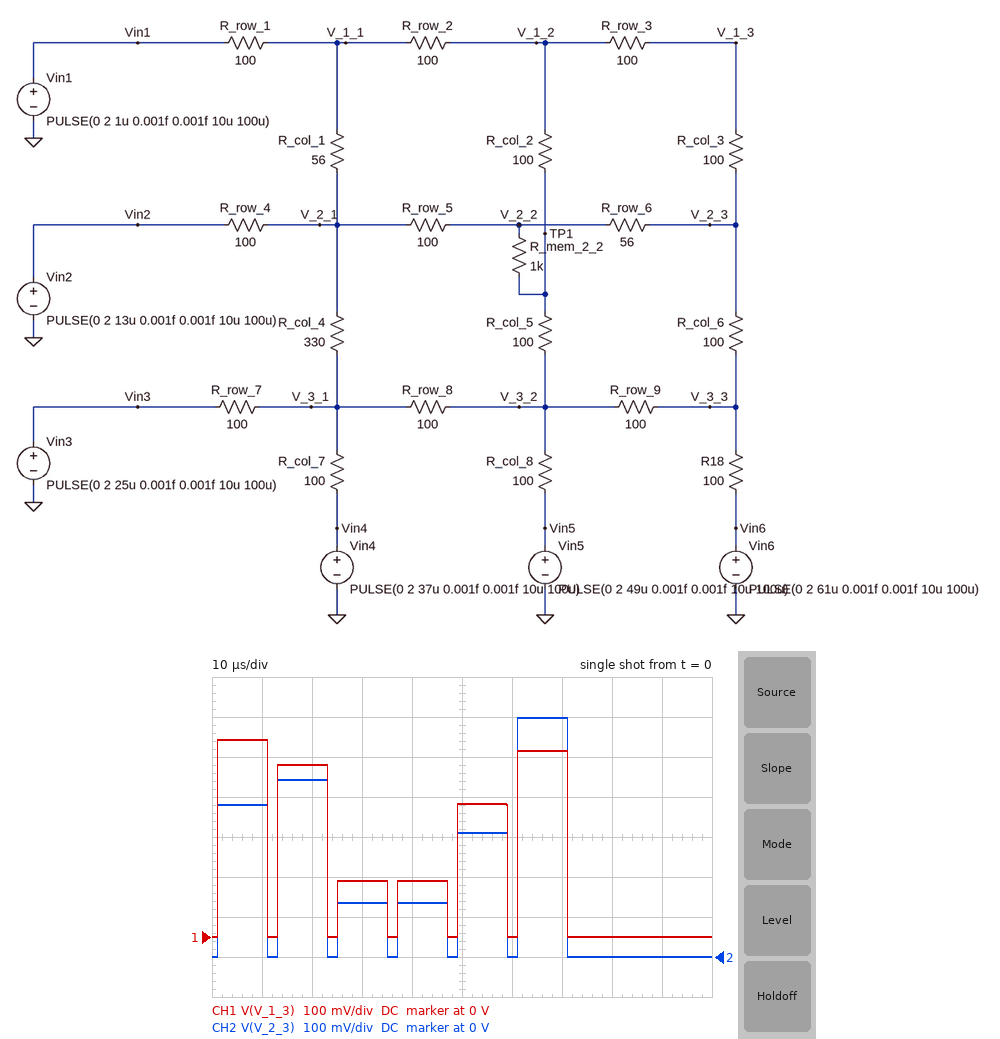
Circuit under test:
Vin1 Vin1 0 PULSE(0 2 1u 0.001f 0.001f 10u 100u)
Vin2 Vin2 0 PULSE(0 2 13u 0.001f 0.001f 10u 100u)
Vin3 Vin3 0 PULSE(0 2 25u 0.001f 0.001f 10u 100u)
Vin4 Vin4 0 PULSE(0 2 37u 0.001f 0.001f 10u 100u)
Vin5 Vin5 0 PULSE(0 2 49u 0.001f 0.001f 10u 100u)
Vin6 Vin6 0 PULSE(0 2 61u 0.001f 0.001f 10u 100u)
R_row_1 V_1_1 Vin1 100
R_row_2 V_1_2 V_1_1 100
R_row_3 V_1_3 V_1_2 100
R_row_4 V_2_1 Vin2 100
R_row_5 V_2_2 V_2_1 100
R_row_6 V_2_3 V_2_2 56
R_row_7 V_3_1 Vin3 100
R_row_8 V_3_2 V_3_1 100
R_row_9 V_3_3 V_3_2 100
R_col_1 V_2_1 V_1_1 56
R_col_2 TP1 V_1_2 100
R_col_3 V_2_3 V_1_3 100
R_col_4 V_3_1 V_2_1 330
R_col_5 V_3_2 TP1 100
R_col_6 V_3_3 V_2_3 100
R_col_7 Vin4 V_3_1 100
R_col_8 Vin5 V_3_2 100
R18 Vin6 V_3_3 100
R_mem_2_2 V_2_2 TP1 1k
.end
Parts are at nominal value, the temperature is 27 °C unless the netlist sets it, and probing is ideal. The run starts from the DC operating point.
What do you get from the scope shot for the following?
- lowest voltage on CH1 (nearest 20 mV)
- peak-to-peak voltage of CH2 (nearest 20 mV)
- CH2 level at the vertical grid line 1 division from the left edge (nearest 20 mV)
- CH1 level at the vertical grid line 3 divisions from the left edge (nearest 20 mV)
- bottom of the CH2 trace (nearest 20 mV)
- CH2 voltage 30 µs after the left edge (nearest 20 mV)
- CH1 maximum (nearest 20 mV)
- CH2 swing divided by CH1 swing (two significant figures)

0 V
600 mV
380 mV
140 mV
0 V
140 mV
500 mV
1.2
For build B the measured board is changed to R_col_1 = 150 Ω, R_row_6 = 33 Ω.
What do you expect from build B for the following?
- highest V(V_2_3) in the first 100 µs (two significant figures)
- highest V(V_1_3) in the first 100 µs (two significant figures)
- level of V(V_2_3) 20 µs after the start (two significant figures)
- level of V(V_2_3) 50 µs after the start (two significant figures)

580 mV
520 mV
490 mV
300 mV
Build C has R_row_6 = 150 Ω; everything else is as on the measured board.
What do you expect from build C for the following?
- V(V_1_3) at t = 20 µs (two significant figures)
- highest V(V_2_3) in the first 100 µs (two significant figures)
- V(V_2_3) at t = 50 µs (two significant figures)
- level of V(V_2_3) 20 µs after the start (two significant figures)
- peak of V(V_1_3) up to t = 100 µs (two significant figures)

390 mV
660 mV
330 mV
380 mV
500 mV
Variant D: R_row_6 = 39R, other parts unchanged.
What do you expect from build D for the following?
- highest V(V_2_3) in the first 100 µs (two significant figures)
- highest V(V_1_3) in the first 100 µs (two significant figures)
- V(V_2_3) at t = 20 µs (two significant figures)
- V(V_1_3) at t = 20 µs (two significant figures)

580 mV
500 mV
460 mV
440 mV
